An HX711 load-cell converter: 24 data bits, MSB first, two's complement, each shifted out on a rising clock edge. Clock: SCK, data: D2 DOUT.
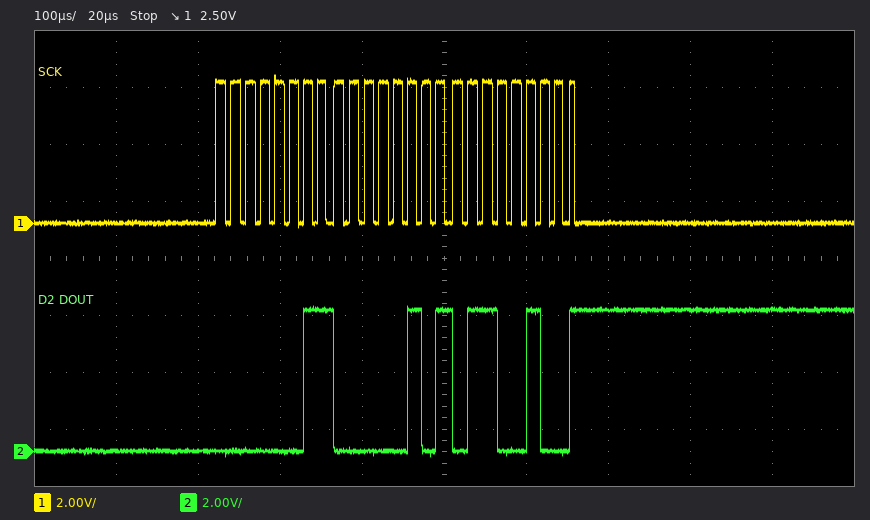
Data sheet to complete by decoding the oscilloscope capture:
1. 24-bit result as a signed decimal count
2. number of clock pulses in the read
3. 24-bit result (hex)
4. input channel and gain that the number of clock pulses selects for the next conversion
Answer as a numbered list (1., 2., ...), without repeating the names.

1. 197988
2. 25
3. 0x030564
4. channel A, gain 128
